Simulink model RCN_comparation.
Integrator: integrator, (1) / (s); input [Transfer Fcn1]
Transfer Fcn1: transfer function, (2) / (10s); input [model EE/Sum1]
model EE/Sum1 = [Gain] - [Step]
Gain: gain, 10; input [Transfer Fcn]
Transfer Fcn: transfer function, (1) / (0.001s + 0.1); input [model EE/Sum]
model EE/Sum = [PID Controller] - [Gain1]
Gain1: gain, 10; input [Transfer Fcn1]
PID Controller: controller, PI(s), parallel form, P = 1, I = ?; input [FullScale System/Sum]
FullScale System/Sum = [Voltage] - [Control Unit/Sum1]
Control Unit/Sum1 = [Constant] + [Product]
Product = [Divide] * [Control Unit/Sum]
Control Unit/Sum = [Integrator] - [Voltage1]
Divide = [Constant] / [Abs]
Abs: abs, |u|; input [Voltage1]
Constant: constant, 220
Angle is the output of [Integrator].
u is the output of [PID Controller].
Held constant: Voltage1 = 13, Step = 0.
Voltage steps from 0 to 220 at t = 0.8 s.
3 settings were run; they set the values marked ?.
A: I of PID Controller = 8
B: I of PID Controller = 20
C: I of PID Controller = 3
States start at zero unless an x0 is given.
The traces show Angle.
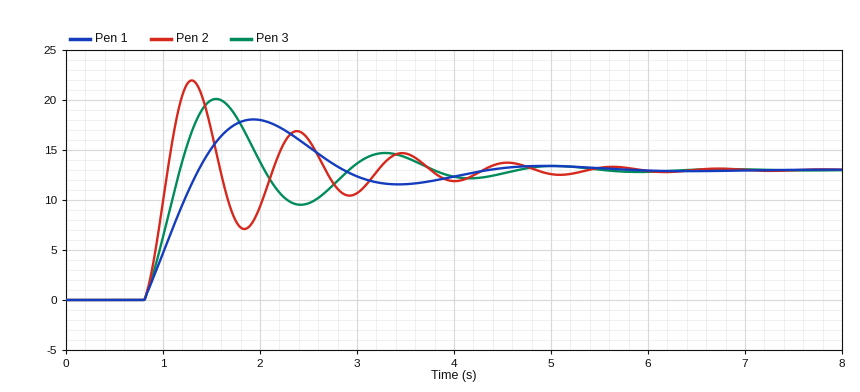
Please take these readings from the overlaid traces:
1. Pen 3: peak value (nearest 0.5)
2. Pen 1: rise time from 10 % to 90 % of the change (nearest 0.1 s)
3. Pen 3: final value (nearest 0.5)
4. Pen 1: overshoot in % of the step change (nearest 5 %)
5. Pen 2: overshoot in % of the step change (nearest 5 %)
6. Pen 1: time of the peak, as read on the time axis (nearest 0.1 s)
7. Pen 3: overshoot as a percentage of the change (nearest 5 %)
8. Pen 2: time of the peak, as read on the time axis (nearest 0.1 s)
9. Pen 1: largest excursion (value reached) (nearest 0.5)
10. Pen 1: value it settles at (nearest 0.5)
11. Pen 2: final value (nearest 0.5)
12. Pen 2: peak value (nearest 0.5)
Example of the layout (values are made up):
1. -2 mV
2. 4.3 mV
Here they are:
1. 20.0
2. 0.4 s
3. 13.0
4. 40 %
5. 70 %
6. 1.9 s
7. 55 %
8. 1.3 s
9. 18.0
10. 13.0
11. 13.0
12. 22.0
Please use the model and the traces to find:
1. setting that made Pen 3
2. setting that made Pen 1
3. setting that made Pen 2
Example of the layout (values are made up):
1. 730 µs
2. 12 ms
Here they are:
1. A
2. C
3. B
